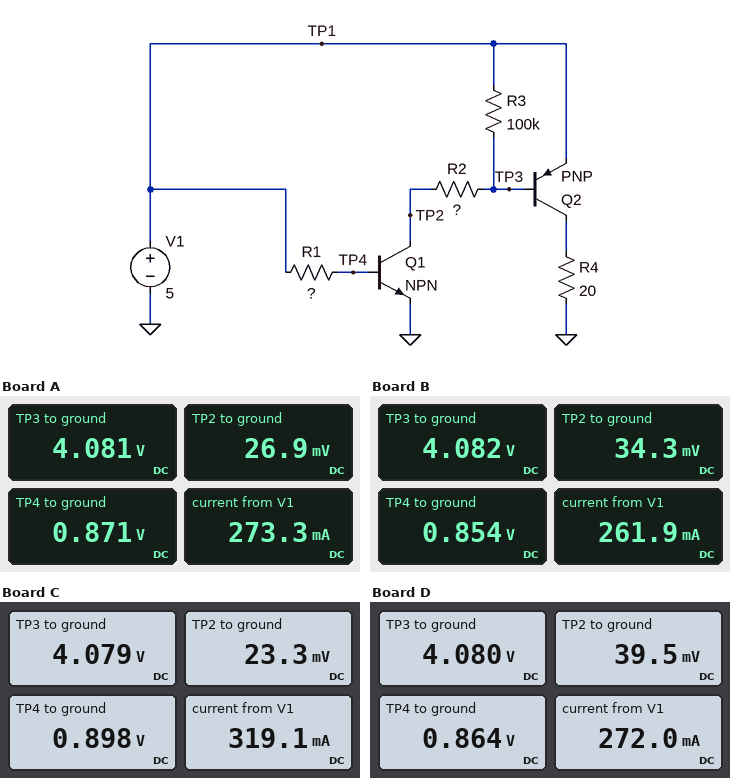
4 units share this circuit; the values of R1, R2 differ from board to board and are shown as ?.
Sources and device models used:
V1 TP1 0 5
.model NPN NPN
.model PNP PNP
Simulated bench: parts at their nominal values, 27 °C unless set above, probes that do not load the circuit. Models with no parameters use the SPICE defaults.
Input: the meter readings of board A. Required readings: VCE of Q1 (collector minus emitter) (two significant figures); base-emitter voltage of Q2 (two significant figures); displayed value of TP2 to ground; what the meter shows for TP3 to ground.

27 mV
-920 mV
26.9 mV
4.081 V
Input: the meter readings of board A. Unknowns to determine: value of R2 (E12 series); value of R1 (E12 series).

330 Ω
270 Ω
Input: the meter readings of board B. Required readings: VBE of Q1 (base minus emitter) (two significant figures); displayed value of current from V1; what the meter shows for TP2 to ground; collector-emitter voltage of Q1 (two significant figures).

850 mV
261.9 mA
34.3 mV
34 mV
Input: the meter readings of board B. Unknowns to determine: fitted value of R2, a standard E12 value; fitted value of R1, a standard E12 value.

390 Ω
680 Ω
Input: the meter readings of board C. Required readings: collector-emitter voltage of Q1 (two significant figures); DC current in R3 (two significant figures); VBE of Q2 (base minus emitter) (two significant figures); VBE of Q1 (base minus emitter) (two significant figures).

23 mV
9.2 µA
-920 mV
900 mV
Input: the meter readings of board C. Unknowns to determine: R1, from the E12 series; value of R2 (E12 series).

82 Ω
180 Ω
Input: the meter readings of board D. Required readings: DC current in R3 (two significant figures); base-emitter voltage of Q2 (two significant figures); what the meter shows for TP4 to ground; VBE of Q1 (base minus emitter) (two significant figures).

9.2 µA
-920 mV
0.864 V
860 mV
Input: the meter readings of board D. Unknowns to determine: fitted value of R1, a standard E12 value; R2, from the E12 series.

560 Ω
220 Ω
